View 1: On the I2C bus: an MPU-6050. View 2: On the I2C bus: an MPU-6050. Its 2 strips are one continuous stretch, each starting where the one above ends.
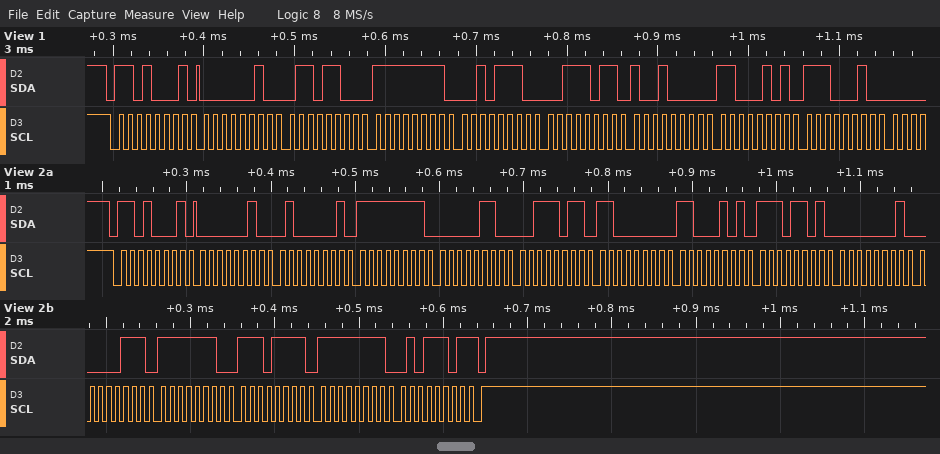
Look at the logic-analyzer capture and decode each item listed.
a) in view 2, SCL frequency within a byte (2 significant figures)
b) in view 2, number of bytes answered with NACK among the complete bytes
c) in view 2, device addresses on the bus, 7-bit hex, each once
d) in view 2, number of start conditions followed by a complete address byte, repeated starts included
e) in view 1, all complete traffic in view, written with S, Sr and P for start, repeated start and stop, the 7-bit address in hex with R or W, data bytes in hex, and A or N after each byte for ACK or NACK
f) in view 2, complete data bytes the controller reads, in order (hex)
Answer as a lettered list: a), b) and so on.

a) 100 kHz
b) 1
c) 0x68
d) 1
e) S 68R A 02 A 6C A FF A 2E A 3B A 90 A C5 A E2 A
f) 02 41 FF 06 3B C0 C5 ED 01 07 FE EF FF 5D
